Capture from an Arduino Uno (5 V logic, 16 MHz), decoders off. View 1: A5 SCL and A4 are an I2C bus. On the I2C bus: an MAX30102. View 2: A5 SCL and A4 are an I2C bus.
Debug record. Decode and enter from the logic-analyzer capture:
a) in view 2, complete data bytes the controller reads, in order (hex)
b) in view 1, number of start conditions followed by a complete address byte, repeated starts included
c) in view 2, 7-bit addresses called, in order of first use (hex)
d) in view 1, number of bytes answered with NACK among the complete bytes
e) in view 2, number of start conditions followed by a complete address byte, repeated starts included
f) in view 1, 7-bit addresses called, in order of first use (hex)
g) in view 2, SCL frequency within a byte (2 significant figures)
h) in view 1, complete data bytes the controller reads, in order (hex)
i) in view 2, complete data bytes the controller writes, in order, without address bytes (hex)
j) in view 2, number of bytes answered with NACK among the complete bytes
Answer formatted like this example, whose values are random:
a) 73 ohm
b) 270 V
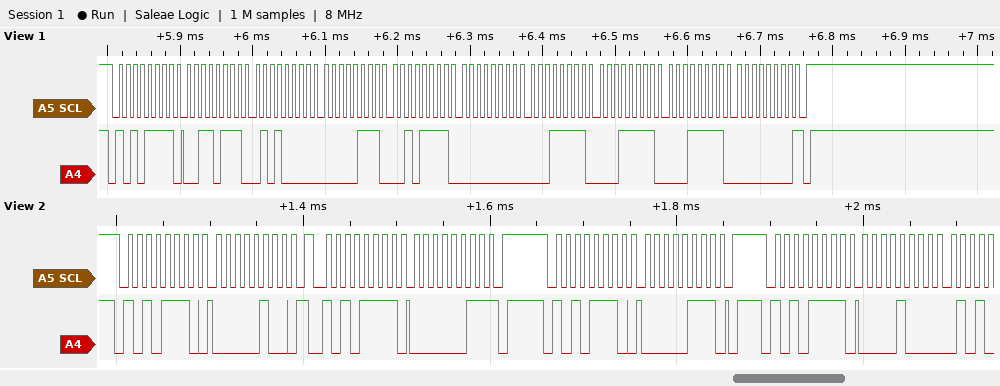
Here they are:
a) 03 08
b) 1
c) 0x57
d) 1
e) 4
f) 0x57
g) 100 kHz
h) 37 50 07 2F 00 1F 1F 1F 00
i) 04 07
j) 1
